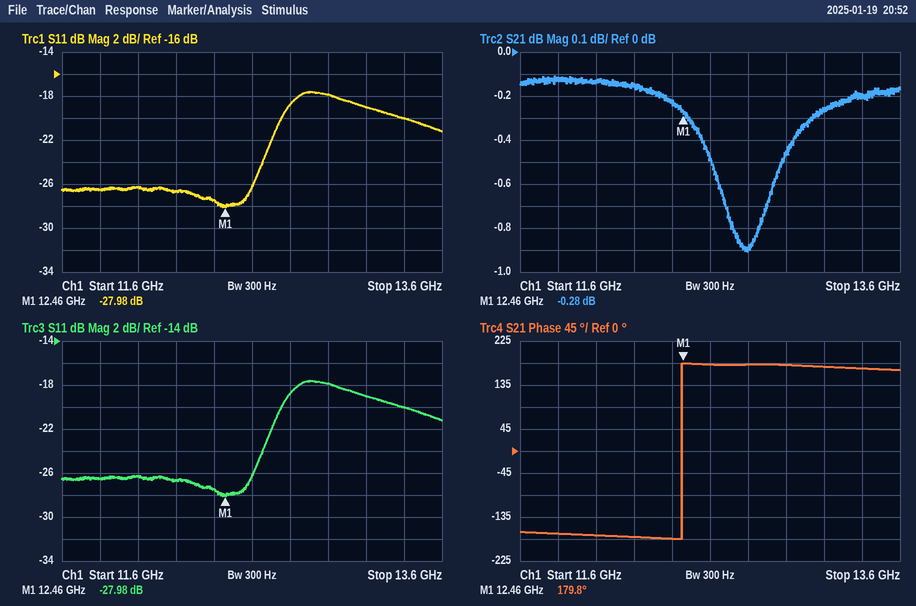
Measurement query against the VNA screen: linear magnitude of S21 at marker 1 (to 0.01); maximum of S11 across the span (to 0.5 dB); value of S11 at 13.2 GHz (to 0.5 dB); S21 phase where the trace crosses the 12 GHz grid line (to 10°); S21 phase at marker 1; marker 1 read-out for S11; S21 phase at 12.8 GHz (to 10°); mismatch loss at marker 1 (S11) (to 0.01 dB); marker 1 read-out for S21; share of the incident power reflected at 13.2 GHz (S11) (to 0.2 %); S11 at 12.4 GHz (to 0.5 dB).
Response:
0.97
-17.5 dB
-19.0 dB
-170°
179.8°
-27.98 dB
180°
0.01 dB
-0.28 dB
1.2 %
-27.5 dB
